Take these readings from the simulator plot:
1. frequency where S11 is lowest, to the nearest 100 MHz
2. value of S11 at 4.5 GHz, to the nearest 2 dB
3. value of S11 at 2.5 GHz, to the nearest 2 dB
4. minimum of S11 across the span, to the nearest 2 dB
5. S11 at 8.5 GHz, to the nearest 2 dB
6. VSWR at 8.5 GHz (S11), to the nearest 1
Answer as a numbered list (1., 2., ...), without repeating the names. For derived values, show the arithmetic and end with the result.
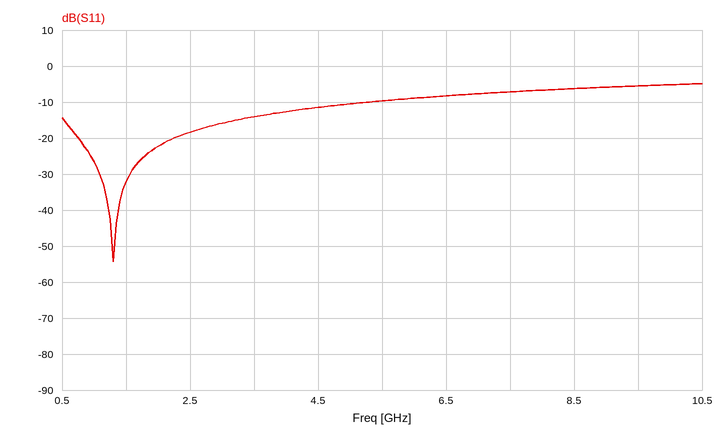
1. 1.3 GHz
2. -12 dB
3. -18 dB
4. -54 dB
5. -6 dB
6. |Γ| = 10^(-6/20) = 0.5012; VSWR = (1 + 0.5012)/(1 − 0.5012) ≈ 3
